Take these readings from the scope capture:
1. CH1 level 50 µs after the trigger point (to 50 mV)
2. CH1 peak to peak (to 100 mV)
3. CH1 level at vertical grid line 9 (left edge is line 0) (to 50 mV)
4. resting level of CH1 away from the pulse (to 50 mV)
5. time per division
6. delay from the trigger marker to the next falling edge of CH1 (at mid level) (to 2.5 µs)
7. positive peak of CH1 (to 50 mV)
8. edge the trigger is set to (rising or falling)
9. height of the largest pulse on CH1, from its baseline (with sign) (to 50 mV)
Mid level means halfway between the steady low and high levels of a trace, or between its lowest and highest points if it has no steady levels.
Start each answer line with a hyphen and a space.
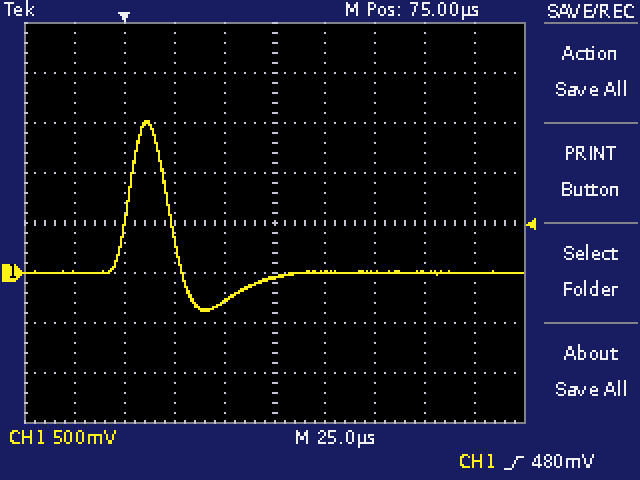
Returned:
- -300 mV
- 1.90 V
- 0 mV
- 0 mV
- 25 µs
- 22.5 µs
- 1.50 V
- rising
- +1.50 V
